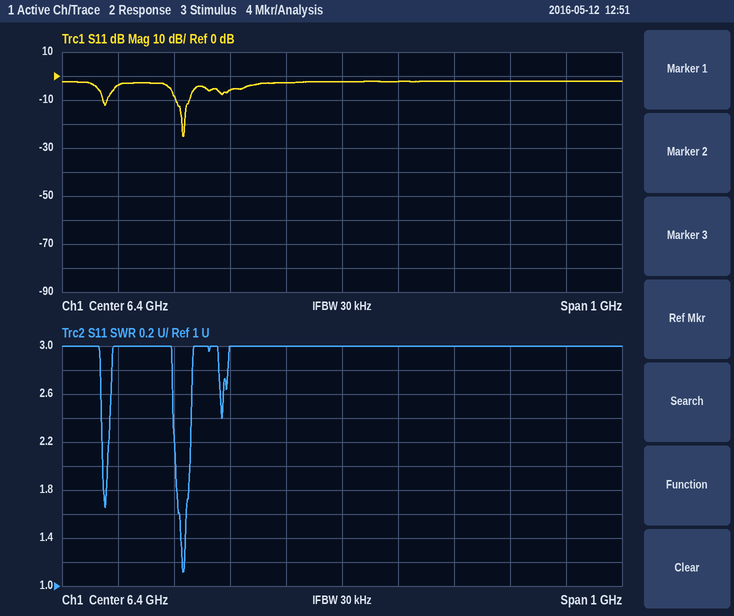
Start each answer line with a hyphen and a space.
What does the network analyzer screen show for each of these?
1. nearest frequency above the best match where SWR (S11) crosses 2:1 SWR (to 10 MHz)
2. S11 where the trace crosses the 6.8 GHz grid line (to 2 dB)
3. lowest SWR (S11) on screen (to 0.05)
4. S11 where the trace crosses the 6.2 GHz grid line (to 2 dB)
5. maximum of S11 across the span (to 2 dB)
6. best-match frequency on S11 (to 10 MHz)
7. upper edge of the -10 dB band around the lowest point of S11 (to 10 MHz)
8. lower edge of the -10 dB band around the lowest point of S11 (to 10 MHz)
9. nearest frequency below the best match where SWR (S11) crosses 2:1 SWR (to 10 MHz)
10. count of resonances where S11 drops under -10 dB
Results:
- 6.13 GHz
- -2 dB
- 1.10
- -6 dB
- -2 dB
- 6.12 GHz
- 6.13 GHz
- 6.10 GHz
- 6.10 GHz
- 2
